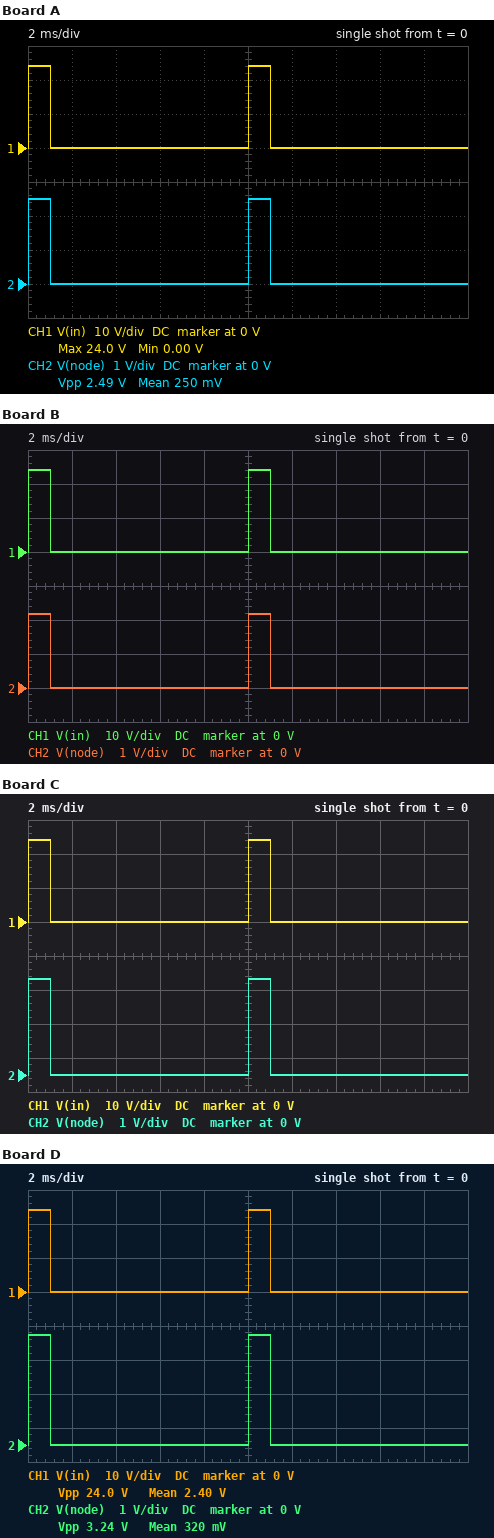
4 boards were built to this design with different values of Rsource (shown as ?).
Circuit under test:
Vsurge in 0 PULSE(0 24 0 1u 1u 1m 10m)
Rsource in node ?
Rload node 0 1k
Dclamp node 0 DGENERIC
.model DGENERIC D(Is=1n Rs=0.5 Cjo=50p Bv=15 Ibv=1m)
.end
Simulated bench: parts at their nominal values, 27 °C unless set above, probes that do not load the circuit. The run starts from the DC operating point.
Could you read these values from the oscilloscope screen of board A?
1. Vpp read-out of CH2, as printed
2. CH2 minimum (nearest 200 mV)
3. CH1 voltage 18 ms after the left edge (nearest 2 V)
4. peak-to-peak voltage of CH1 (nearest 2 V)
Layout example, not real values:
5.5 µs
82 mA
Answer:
2.49 V
0 V
0 V
24 V
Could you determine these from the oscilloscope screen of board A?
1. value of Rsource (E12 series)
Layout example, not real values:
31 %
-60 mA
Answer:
5.6 Ω
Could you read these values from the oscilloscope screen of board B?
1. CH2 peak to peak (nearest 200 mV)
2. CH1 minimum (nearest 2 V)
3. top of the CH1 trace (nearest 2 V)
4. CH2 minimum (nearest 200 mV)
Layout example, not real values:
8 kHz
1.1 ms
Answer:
2.2 V
0 V
24 V
0 V
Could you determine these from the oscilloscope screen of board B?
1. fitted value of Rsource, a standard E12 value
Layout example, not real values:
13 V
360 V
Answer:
6.8 Ω
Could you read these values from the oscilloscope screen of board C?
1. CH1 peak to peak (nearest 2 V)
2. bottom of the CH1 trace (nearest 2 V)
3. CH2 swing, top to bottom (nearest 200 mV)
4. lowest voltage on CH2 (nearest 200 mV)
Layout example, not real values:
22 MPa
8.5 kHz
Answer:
24 V
0 V
2.8 V
0 V
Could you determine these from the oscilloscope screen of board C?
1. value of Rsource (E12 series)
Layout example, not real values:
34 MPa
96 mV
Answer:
4.7 Ω
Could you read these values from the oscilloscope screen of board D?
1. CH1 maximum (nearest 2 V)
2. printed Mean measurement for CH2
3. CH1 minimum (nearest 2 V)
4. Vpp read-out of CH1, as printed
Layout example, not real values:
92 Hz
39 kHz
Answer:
24 V
320 mV
0 V
24.0 V
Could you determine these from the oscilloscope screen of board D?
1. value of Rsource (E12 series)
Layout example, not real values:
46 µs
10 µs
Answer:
3.9 Ω
